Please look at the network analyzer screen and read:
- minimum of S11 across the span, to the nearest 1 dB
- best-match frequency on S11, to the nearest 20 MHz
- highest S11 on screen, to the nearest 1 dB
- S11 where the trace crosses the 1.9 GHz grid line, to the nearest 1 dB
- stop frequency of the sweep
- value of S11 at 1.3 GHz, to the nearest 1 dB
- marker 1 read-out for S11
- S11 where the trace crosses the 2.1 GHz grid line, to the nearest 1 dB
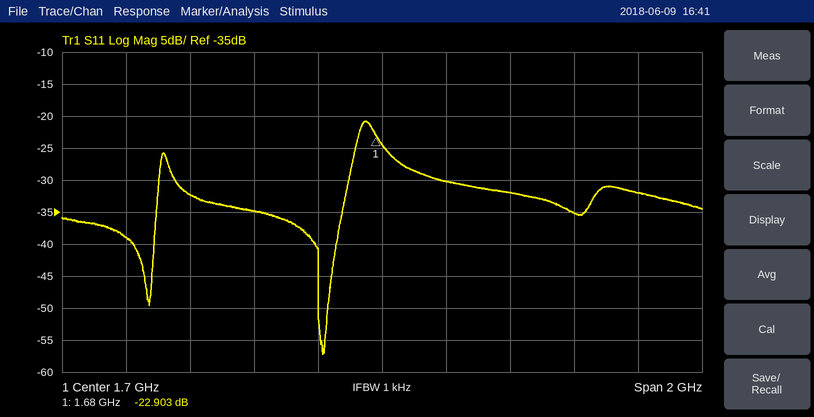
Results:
-57 dB
1.52 GHz
-21 dB
-30 dB
2.7 GHz
-35 dB
-22.903 dB
-32 dB
